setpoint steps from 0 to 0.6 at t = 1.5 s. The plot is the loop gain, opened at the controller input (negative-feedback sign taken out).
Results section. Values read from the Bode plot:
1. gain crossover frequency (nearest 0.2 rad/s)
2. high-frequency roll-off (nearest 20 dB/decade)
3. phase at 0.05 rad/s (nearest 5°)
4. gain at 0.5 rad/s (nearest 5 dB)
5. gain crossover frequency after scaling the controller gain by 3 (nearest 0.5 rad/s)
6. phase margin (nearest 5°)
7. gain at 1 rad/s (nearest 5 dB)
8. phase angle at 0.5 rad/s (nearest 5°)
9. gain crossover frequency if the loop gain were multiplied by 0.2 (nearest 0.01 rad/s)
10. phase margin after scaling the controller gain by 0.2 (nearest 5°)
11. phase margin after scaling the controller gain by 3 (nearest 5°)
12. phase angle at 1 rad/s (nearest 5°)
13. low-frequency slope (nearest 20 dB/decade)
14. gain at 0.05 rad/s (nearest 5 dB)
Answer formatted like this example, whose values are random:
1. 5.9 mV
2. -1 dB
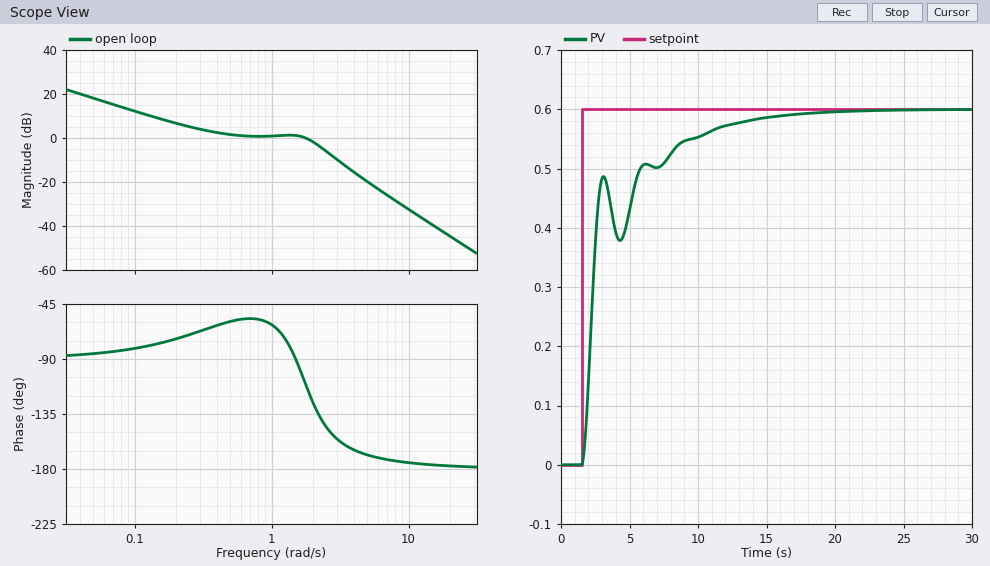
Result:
1. 1.8 rad/s
2. -40 dB/decade
3. -85°
4. 0 dB
5. 3.0 rad/s
6. 70°
7. 0 dB
8. -60°
9. 0.08 rad/s
10. 95°
11. 25°
12. -60°
13. -20 dB/decade
14. 20 dB
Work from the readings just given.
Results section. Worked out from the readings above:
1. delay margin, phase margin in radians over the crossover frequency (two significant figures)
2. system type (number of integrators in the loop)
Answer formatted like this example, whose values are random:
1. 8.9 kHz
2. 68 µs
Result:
1. 0.68 s
2. 1
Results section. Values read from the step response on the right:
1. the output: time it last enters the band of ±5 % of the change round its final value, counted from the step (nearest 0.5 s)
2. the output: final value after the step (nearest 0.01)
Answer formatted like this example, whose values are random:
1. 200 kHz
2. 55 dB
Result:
1. 10.0 s
2. 0.60
